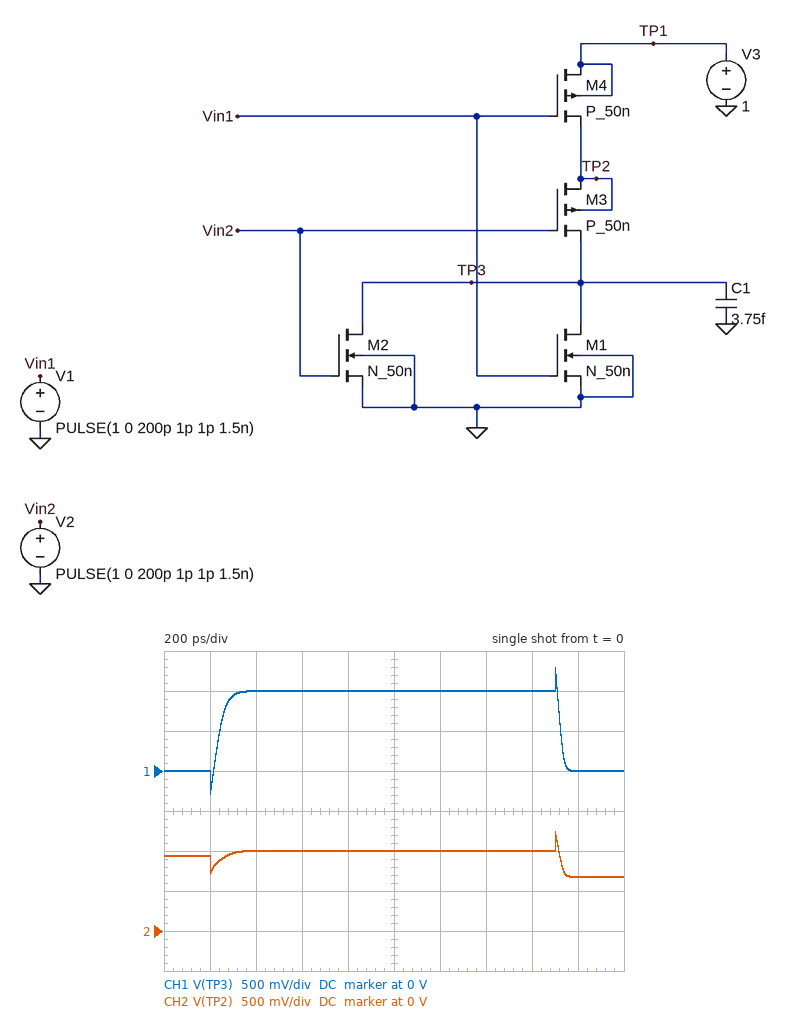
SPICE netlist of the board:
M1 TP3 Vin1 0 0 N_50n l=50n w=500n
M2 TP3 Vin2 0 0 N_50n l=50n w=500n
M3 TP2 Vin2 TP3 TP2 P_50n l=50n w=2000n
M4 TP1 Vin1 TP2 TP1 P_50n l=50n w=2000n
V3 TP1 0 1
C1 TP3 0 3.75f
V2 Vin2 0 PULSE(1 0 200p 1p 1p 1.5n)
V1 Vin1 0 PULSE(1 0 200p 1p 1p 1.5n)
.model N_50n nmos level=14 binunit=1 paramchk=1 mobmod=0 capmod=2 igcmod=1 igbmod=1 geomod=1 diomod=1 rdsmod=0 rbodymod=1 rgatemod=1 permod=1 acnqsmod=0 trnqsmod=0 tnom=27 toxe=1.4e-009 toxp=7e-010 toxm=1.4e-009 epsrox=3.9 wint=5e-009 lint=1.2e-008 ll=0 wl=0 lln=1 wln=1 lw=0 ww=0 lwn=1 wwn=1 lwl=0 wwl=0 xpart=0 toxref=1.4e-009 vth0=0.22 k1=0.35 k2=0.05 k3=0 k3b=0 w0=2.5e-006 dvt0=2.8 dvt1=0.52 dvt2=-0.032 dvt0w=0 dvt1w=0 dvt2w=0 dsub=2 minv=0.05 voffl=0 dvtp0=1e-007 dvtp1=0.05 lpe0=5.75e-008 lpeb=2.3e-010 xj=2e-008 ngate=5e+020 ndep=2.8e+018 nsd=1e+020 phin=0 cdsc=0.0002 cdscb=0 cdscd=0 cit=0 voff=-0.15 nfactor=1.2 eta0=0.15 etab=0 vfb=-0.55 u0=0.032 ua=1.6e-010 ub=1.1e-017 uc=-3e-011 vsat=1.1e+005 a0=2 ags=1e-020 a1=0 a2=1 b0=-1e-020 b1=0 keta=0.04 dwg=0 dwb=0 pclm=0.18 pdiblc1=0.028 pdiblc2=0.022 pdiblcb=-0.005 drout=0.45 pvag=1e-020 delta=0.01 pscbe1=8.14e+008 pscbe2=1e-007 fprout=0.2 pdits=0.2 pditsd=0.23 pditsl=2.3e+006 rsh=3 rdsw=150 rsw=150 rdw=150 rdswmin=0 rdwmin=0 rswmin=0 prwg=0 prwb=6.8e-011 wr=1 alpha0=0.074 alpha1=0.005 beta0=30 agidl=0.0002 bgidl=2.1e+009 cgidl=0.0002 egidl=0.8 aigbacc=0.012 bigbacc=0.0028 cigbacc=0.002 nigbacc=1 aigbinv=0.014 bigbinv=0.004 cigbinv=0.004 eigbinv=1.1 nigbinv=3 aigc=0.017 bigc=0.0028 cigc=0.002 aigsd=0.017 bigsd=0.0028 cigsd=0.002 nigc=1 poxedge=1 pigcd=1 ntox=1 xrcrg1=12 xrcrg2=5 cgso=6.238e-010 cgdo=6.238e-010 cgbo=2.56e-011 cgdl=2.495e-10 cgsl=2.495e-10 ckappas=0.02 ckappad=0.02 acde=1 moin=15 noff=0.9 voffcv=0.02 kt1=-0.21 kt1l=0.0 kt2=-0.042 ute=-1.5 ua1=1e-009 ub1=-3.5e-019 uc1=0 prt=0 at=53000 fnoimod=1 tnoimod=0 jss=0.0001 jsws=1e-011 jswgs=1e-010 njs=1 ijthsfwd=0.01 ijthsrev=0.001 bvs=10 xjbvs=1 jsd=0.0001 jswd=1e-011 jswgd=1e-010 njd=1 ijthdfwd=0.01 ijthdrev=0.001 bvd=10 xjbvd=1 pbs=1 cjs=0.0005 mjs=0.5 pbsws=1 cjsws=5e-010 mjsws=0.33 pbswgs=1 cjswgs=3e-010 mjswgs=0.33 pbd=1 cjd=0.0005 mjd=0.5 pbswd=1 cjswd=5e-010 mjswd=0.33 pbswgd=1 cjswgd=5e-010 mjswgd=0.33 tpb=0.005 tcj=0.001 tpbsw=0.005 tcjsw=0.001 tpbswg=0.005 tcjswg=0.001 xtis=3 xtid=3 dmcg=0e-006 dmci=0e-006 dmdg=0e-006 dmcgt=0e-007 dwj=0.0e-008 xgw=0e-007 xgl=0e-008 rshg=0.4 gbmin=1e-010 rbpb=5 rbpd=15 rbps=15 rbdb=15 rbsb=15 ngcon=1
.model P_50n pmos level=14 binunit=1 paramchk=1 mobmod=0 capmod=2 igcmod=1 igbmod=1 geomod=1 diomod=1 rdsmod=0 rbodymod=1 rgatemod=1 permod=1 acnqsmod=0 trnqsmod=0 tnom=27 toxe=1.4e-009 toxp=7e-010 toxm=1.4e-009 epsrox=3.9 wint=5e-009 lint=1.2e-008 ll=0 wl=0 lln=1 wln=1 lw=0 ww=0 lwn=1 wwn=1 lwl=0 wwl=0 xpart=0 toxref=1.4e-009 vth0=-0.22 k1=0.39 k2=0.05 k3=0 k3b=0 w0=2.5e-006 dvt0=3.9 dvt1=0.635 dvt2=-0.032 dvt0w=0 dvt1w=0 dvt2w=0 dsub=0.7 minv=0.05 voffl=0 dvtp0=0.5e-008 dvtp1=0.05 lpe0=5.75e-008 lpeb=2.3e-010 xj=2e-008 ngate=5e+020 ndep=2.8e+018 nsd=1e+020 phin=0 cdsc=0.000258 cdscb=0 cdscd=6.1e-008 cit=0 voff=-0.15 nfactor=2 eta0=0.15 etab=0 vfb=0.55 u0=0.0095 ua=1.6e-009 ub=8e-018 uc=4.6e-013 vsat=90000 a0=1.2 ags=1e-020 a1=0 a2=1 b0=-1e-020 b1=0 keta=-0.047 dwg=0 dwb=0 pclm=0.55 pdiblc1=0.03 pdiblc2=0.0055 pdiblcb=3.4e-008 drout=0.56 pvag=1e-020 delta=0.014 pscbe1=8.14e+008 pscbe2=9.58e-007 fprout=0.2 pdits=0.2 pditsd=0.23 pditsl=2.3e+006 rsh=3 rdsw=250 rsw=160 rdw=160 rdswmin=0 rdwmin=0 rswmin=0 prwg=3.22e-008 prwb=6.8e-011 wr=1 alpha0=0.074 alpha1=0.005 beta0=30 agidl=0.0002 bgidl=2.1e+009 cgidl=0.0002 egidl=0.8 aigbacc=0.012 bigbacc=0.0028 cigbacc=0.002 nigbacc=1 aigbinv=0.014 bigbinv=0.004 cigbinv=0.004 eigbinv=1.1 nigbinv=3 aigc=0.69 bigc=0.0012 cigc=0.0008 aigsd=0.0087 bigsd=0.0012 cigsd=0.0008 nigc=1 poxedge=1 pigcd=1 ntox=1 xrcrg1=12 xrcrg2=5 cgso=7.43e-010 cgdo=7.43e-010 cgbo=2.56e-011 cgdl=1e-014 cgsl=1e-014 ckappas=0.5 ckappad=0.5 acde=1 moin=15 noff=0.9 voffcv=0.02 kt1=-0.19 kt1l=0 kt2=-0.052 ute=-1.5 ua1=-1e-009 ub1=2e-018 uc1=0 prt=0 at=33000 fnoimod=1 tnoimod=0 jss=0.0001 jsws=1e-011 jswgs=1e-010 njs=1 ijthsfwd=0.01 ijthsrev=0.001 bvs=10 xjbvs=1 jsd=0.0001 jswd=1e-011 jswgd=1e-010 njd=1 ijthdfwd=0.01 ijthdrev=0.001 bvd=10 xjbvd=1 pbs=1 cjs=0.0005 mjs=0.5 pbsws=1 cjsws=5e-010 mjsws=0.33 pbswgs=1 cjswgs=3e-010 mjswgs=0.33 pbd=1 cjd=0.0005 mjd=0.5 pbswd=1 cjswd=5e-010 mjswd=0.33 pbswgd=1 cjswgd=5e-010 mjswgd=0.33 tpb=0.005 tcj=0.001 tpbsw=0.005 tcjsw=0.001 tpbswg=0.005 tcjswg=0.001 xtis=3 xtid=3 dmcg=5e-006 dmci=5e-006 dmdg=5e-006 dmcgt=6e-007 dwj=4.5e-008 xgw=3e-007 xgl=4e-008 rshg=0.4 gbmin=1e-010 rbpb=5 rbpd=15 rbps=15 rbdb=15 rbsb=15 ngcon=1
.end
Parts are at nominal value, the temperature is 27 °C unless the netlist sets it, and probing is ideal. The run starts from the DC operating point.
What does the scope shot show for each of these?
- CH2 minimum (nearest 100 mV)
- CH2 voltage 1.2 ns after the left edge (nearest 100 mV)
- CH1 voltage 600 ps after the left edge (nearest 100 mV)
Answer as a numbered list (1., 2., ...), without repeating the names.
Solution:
1. 700 mV
2. 1.0 V
3. 1.0 V
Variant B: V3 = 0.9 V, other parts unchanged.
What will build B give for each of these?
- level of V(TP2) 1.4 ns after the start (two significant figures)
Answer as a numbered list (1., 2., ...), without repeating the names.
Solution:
1. 900 mV
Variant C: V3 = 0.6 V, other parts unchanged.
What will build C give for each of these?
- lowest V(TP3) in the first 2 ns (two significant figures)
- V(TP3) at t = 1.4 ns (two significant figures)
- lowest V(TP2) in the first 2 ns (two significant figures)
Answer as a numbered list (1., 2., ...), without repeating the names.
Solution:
1. -280 mV
2. 600 mV
3. 430 mV
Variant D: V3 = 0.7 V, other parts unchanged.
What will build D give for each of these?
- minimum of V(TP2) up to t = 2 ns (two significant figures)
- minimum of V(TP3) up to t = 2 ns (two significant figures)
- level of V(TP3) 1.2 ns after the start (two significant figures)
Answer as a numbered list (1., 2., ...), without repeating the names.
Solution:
1. 490 mV
2. -280 mV
3. 700 mV
